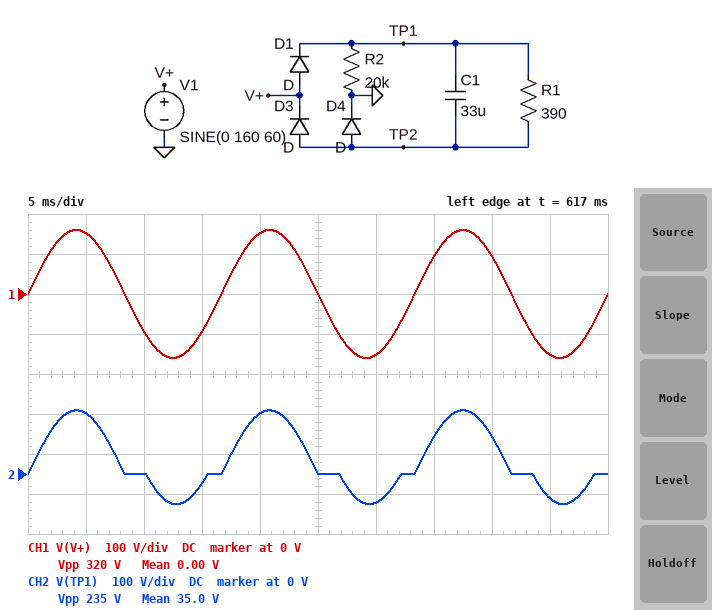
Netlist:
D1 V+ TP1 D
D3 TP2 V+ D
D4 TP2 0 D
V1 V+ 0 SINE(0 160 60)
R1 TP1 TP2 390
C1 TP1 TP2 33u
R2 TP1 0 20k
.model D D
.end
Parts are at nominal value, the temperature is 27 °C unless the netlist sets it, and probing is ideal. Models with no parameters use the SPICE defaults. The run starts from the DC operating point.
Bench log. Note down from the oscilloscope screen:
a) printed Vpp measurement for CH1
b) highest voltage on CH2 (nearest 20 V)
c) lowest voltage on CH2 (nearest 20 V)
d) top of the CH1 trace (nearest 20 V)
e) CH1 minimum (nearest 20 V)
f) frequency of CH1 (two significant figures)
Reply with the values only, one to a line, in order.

320 V
160 V
-80 V
160 V
-160 V
60 Hz
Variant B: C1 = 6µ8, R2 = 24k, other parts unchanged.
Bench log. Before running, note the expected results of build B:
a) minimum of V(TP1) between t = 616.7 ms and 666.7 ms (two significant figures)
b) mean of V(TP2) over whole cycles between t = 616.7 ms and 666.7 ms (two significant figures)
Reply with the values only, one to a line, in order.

-150 V
-54 V
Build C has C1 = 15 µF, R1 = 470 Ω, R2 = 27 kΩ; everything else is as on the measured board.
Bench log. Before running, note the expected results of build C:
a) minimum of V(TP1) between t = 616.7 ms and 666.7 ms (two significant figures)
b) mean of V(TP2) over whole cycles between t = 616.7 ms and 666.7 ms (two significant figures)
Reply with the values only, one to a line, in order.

-110 V
-62 V
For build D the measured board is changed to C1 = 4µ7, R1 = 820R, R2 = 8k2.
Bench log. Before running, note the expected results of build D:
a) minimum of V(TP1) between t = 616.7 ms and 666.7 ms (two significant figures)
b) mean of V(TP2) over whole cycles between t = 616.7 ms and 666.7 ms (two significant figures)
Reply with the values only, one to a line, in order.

-130 V
-56 V
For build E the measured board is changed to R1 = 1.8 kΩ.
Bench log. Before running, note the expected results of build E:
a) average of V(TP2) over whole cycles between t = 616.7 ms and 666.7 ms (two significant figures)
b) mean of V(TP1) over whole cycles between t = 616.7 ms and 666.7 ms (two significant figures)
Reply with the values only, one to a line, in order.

-93 V
48 V
